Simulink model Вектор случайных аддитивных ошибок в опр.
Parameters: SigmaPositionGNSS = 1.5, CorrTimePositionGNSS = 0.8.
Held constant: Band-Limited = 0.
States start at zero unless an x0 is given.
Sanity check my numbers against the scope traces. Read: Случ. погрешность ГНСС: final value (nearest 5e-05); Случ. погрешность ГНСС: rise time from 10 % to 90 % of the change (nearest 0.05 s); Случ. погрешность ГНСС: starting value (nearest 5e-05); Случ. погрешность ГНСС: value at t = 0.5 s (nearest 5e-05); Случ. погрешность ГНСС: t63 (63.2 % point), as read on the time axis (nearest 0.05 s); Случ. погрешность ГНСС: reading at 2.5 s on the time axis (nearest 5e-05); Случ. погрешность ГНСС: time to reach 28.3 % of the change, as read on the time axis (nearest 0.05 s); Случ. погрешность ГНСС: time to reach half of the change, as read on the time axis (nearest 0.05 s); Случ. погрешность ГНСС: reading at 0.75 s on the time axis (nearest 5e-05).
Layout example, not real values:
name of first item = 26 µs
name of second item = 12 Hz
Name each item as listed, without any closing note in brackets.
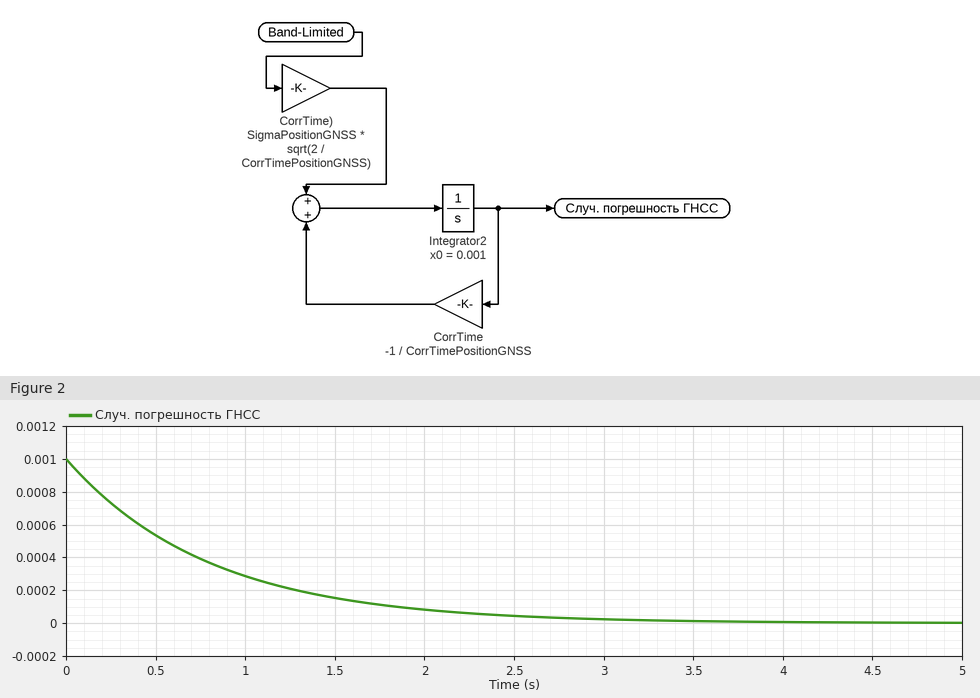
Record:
Случ. погрешность ГНСС: final value = 0.00000
Случ. погрешность ГНСС: rise time from 10 % to 90 % of the change = 1.75 s
Случ. погрешность ГНСС: starting value = 0.00100
Случ. погрешность ГНСС: value at t = 0.5 s = 0.00055
Случ. погрешность ГНСС: t63 (63.2 % point), as read on the time axis = 0.80 s
Случ. погрешность ГНСС: reading at 2.5 s on the time axis = 0.00005
Случ. погрешность ГНСС: time to reach 28.3 % of the change, as read on the time axis = 0.25 s
Случ. погрешность ГНСС: time to reach half of the change, as read on the time axis = 0.55 s
Случ. погрешность ГНСС: reading at 0.75 s on the time axis = 0.00040
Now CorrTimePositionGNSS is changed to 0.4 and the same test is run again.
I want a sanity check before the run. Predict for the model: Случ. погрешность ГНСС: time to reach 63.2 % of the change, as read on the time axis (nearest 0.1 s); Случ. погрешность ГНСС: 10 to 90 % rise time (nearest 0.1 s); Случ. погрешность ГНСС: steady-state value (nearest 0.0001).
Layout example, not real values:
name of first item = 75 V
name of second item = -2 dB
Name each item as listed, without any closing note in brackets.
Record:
Случ. погрешность ГНСС: time to reach 63.2 % of the change, as read on the time axis = 0.4 s
Случ. погрешность ГНСС: 10 to 90 % rise time = 0.9 s
Случ. погрешность ГНСС: steady-state value = 0.0000
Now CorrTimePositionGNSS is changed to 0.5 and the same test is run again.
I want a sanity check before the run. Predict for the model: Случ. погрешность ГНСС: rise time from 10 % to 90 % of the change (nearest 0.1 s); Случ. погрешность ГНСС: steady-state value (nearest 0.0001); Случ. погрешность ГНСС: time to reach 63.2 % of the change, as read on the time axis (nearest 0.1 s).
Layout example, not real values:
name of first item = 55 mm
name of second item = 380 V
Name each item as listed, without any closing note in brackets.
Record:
Случ. погрешность ГНСС: rise time from 10 % to 90 % of the change = 1.1 s
Случ. погрешность ГНСС: steady-state value = 0.0000
Случ. погрешность ГНСС: time to reach 63.2 % of the change, as read on the time axis = 0.5 s
